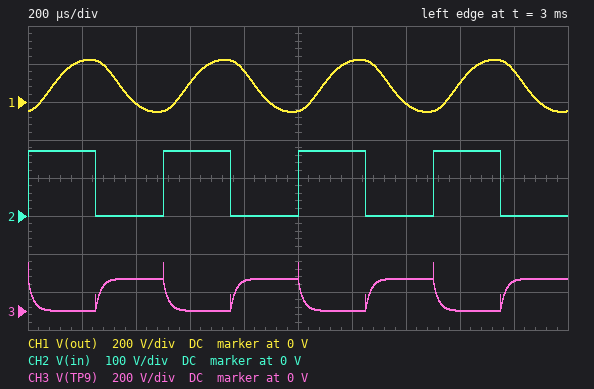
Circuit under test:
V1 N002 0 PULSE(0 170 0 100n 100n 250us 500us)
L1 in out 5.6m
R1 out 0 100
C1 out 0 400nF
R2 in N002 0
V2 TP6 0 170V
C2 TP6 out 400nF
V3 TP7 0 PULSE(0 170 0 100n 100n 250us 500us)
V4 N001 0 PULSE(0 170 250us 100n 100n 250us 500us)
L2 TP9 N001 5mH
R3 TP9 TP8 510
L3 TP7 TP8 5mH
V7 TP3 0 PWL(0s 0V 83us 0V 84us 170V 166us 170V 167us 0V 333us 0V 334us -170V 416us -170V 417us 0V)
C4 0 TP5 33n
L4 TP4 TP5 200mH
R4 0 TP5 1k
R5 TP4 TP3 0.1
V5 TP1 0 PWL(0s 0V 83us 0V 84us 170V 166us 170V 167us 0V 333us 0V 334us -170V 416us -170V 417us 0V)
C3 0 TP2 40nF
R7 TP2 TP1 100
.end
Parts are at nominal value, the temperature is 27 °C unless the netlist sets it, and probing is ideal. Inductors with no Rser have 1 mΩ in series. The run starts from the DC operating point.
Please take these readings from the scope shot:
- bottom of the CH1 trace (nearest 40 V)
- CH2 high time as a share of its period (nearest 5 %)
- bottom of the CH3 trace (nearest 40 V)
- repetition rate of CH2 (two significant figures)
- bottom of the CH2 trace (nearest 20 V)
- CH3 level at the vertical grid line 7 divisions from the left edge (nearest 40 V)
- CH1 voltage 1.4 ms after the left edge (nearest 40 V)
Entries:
-40 V
50 %
0 V
2.0 kHz
0 V
160 V
0 V
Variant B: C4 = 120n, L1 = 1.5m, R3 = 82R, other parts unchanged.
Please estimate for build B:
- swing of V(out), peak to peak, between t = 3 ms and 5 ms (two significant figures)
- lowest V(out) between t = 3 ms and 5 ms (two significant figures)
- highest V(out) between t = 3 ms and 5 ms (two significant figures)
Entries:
310 V
-71 V
240 V
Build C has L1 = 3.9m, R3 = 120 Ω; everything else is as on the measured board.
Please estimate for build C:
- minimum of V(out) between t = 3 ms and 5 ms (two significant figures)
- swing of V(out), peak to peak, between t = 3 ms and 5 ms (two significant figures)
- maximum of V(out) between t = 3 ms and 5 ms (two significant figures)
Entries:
-62 V
290 V
230 V
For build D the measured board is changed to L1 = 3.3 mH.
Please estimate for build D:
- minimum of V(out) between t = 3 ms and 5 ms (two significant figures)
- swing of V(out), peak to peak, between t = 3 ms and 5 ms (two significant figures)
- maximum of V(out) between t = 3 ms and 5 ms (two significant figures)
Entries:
-63 V
300 V
230 V
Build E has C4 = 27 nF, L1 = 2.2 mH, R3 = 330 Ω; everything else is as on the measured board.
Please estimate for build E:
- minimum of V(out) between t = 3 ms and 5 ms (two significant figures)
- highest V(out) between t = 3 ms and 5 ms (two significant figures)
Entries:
-63 V
230 V
